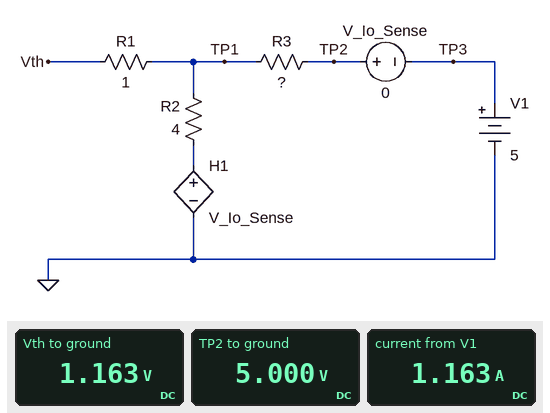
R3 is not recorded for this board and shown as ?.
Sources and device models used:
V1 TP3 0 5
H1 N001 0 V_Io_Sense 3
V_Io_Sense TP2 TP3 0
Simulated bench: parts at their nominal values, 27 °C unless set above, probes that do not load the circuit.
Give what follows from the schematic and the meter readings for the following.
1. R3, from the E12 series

3.3 Ω
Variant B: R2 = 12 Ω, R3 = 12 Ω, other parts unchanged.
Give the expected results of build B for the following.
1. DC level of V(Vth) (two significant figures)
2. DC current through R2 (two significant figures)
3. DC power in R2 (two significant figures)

2.1 V
240 mA
680 mW
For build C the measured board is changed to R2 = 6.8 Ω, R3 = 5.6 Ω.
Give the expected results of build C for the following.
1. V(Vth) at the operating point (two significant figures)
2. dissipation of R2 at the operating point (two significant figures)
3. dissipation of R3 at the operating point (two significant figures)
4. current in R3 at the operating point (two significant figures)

2.0 V
1.9 W
1.6 W
530 mA
